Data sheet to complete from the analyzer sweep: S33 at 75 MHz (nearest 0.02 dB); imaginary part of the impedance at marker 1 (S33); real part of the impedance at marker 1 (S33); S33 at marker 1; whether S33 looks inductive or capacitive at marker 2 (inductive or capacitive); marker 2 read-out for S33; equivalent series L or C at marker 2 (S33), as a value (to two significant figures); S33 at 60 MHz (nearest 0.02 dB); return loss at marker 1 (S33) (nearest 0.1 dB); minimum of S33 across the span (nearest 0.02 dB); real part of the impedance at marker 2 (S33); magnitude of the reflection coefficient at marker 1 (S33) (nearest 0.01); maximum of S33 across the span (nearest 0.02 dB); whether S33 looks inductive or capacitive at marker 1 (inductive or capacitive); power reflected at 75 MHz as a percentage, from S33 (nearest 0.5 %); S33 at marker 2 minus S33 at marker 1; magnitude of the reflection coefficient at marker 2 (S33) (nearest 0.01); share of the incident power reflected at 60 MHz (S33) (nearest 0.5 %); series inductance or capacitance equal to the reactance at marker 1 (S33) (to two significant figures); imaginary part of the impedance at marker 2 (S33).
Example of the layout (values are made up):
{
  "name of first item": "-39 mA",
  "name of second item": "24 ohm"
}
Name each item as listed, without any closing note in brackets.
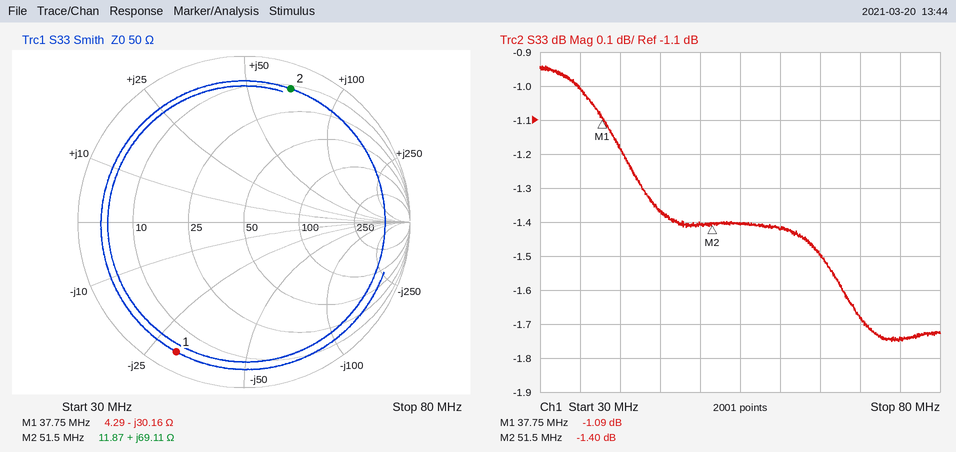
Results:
{
  "S33 at 75 MHz": "-1.74 dB",
  "imaginary part of the impedance at marker 1": "-30.16 Ω",
  "real part of the impedance at marker 1": "4.29 Ω",
  "S33 at marker 1": "-1.09 dB",
  "whether S33 looks inductive or capacitive at marker 2": "inductive",
  "marker 2 read-out for S33": "-1.40 dB",
  "equivalent series L or C at marker 2 (S33), as a value": "210 nH",
  "S33 at 60 MHz": "-1.42 dB",
  "return loss at marker 1 (S33)": "1.1 dB",
  "minimum of S33 across the span": "-1.76 dB",
  "real part of the impedance at marker 2": "11.87 Ω",
  "magnitude of the reflection coefficient at marker 1 (S33)": "0.88",
  "maximum of S33 across the span": "-0.94 dB",
  "whether S33 looks inductive or capacitive at marker 1": "capacitive",
  "power reflected at 75 MHz as a percentage, from S33": "67.0 %",
  "S33 at marker 2 minus S33 at marker 1": "-0.31 dB",
  "magnitude of the reflection coefficient at marker 2 (S33)": "0.85",
  "share of the incident power reflected at 60 MHz (S33)": "72.0 %",
  "series inductance or capacitance equal to the reactance at marker 1 (S33)": "140 pF",
  "imaginary part of the impedance at marker 2": "+69.11 Ω"
}
